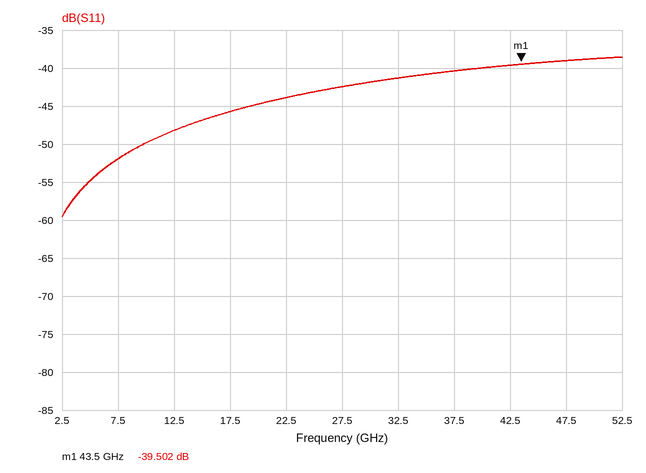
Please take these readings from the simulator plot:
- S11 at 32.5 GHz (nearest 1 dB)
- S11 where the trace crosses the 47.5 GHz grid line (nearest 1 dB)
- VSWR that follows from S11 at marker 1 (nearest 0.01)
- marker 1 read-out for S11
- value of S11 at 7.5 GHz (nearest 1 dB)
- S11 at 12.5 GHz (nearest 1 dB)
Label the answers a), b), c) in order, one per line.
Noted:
a) -41 dB
b) -39 dB
c) 1.02
d) -39.502 dB
e) -52 dB
f) -48 dB
